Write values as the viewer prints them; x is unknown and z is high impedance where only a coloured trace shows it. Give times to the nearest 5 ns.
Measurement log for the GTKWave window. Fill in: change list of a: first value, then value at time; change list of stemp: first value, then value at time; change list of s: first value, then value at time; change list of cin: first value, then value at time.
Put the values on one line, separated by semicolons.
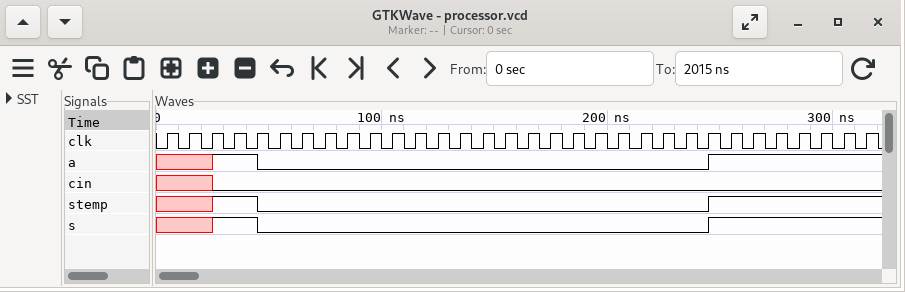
x, 1 at 25 ns, 0 at 45 ns, 1 at 245 ns; x, 1 at 25 ns, 0 at 45 ns, 1 at 245 ns; x, 1 at 25 ns, 0 at 45 ns, 1 at 245 ns; x, 0 at 25 ns
